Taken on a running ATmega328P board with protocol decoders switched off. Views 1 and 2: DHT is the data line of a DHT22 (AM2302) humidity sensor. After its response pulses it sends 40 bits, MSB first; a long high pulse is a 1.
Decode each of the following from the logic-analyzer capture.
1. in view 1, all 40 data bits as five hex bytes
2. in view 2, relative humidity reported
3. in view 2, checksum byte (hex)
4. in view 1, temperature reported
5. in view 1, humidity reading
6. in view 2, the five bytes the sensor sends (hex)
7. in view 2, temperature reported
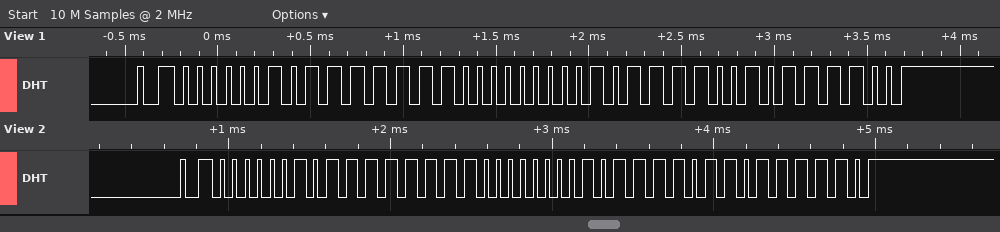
02 FE 00 BC BC
76.7 %
0xBE
18.8 °C
76.6 %
02 FF 00 BD BE
18.9 °C
